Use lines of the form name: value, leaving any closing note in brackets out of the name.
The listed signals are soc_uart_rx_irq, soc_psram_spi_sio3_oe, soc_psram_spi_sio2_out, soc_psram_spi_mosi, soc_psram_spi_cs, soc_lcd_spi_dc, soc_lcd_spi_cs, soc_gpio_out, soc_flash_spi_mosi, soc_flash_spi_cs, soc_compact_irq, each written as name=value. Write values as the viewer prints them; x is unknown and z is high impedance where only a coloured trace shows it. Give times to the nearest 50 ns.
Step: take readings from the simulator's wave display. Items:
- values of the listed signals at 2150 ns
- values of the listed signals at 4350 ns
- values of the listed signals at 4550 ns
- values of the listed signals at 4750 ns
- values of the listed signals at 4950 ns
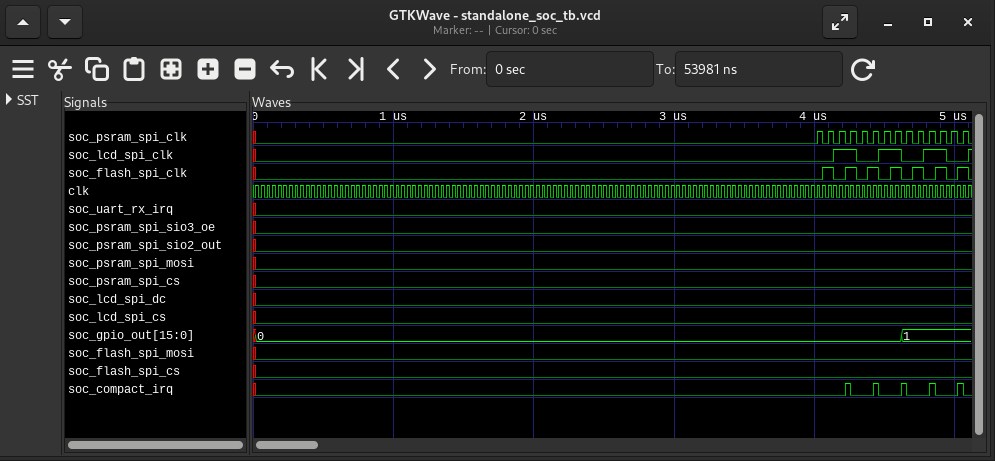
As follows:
values of the listed signals at 2150 ns: soc_uart_rx_irq=0, soc_psram_spi_sio3_oe=0, soc_psram_spi_sio2_out=0, soc_psram_spi_mosi=0, soc_psram_spi_cs=0, soc_lcd_spi_dc=0, soc_lcd_spi_cs=0, soc_gpio_out=0, soc_flash_spi_mosi=0, soc_flash_spi_cs=0, soc_compact_irq=0
values of the listed signals at 4350 ns: soc_uart_rx_irq=0, soc_psram_spi_sio3_oe=0, soc_psram_spi_sio2_out=0, soc_psram_spi_mosi=0, soc_psram_spi_cs=0, soc_lcd_spi_dc=0, soc_lcd_spi_cs=0, soc_gpio_out=0, soc_flash_spi_mosi=0, soc_flash_spi_cs=0, soc_compact_irq=0
values of the listed signals at 4550 ns: soc_uart_rx_irq=0, soc_psram_spi_sio3_oe=0, soc_psram_spi_sio2_out=0, soc_psram_spi_mosi=0, soc_psram_spi_cs=0, soc_lcd_spi_dc=0, soc_lcd_spi_cs=0, soc_gpio_out=0, soc_flash_spi_mosi=0, soc_flash_spi_cs=0, soc_compact_irq=0
values of the listed signals at 4750 ns: soc_uart_rx_irq=0, soc_psram_spi_sio3_oe=0, soc_psram_spi_sio2_out=0, soc_psram_spi_mosi=0, soc_psram_spi_cs=0, soc_lcd_spi_dc=0, soc_lcd_spi_cs=0, soc_gpio_out=1, soc_flash_spi_mosi=0, soc_flash_spi_cs=0, soc_compact_irq=0
values of the listed signals at 4950 ns: soc_uart_rx_irq=0, soc_psram_spi_sio3_oe=0, soc_psram_spi_sio2_out=0, soc_psram_spi_mosi=0, soc_psram_spi_cs=0, soc_lcd_spi_dc=0, soc_lcd_spi_cs=0, soc_gpio_out=1, soc_flash_spi_mosi=0, soc_flash_spi_cs=0, soc_compact_irq=0
